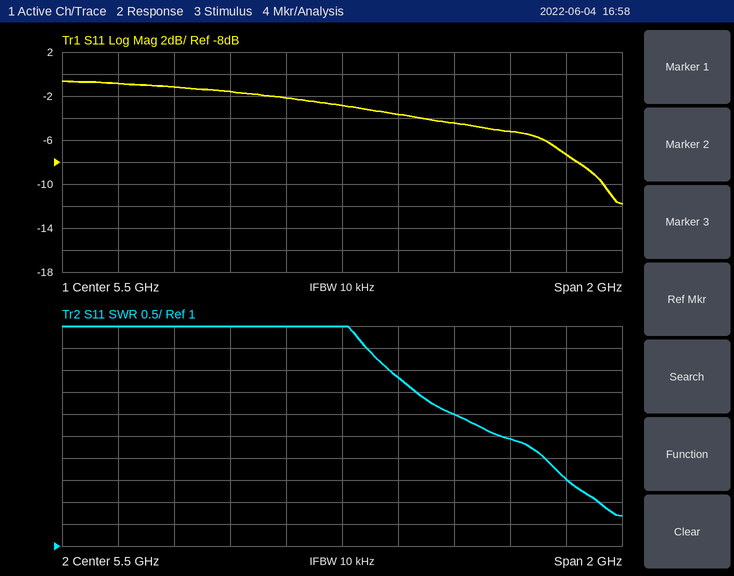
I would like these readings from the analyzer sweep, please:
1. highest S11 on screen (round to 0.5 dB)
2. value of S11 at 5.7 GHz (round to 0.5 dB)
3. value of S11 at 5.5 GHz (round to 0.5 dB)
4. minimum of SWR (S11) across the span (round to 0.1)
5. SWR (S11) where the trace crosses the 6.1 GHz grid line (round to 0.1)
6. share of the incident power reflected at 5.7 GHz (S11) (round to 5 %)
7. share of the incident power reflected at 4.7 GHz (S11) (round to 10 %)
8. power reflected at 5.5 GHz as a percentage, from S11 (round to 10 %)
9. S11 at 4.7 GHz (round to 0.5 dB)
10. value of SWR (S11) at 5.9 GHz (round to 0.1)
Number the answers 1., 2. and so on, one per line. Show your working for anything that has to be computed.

1. -0.5 dB
2. -3.5 dB
3. -3.0 dB
4. 1.7
5. 3.4
6. 10^(-3.5/10) ≈ 45 %
7. 10^(-1/10) ≈ 79.4 %, so 80 % to the nearest 10 %
8. 10^(-3/10) ≈ 50 %
9. -1.0 dB
10. 4.0
